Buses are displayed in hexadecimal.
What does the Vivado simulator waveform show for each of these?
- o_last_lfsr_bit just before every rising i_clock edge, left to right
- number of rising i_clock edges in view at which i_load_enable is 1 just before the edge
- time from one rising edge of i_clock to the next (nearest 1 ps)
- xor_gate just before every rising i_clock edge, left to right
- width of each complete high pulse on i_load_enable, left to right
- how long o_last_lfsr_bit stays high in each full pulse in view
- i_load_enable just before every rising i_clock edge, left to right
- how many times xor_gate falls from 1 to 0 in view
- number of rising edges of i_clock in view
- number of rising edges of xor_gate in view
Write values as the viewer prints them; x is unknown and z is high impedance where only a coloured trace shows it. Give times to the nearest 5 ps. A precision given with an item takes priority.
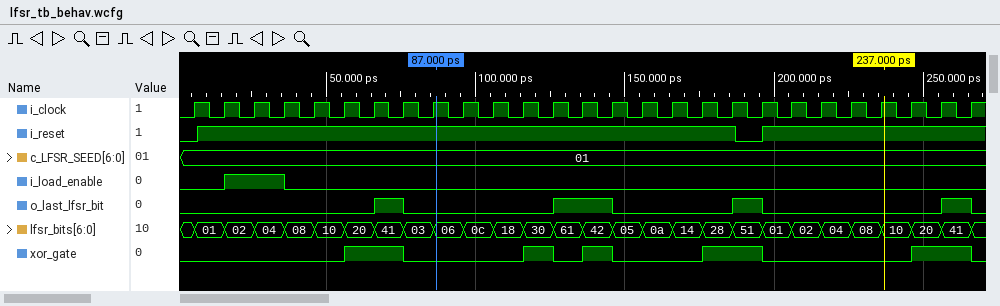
0 0 0 0 0 0 0 1 0 0 0 0 0 1 1 0 0 0 0 1 0 0 0 0 0 0 1
2
10 ps
0 0 0 0 0 0 1 1 0 0 0 0 1 0 1 0 0 0 1 1 0 0 0 0 0 1 1
20 ps
10 ps, 20 ps, 10 ps, 10 ps
0 0 1 1 0 0 0 0 0 0 0 0 0 0 0 0 0 0 0 0 0 0 0 0 0 0 0
5
27
5
